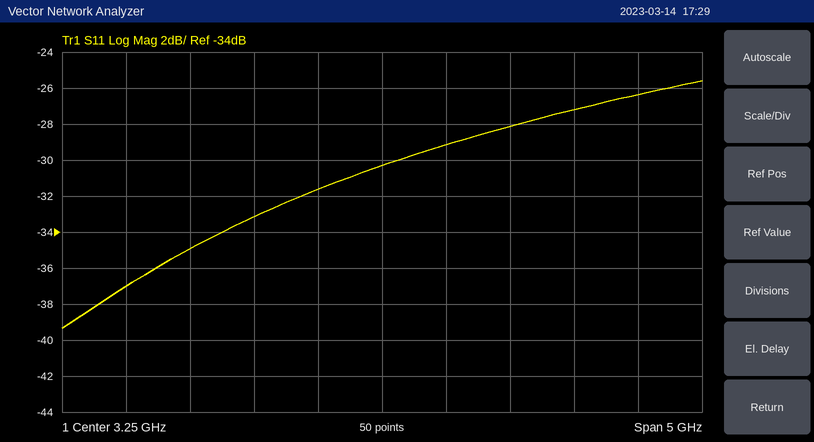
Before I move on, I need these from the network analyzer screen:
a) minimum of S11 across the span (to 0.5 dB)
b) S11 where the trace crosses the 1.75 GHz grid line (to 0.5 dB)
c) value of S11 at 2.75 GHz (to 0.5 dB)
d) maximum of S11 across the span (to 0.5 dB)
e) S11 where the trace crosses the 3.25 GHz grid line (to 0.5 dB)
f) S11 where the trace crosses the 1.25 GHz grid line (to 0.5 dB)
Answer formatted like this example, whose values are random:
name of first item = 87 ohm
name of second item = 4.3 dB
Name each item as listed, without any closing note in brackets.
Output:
minimum of S11 across the span = -39.5 dB
S11 where the trace crosses the 1.75 GHz grid line = -35.0 dB
value of S11 at 2.75 GHz = -31.5 dB
maximum of S11 across the span = -25.5 dB
S11 where the trace crosses the 3.25 GHz grid line = -30.5 dB
S11 where the trace crosses the 1.25 GHz grid line = -37.0 dB
